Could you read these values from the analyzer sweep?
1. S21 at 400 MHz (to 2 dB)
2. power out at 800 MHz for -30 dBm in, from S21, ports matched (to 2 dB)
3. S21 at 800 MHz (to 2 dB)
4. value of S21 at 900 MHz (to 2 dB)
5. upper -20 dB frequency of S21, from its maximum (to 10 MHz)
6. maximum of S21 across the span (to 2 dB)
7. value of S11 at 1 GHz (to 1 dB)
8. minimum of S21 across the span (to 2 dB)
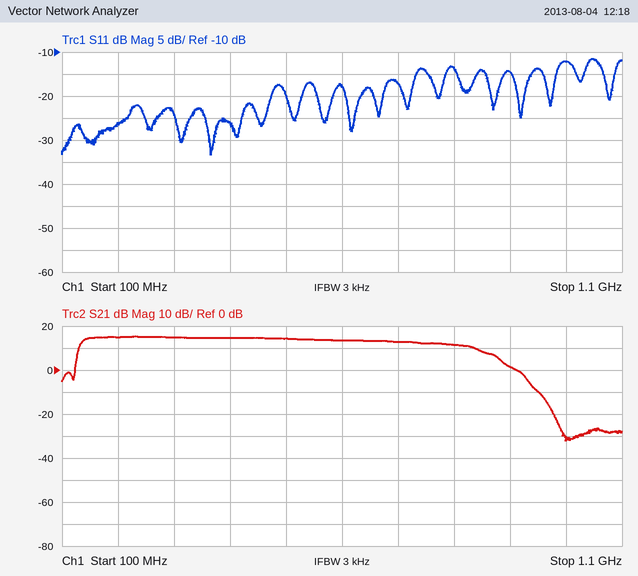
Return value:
14 dB
-18 dBm
12 dB
2 dB
930 MHz
16 dB
-12 dB
-32 dB
